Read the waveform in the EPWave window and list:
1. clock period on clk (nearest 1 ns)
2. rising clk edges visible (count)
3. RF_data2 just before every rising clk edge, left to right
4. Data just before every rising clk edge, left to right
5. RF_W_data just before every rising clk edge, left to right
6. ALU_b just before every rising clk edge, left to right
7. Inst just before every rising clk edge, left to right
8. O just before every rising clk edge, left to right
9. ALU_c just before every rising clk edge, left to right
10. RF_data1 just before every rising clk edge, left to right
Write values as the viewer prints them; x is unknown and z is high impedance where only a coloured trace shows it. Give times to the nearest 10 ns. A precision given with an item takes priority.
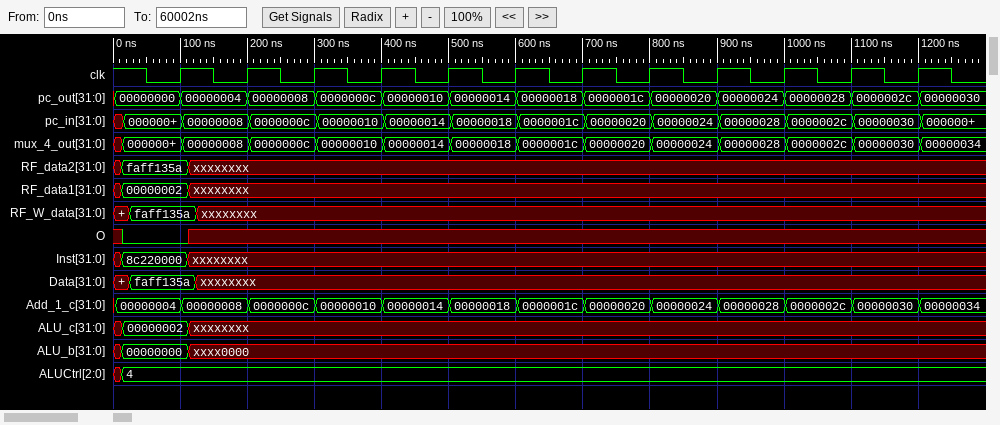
100 ns
12
faff135a, xxxxxxxx, xxxxxxxx, xxxxxxxx, xxxxxxxx, xxxxxxxx, xxxxxxxx, xxxxxxxx, xxxxxxxx, xxxxxxxx, xxxxxxxx, xxxxxxxx
faff135a, xxxxxxxx, xxxxxxxx, xxxxxxxx, xxxxxxxx, xxxxxxxx, xxxxxxxx, xxxxxxxx, xxxxxxxx, xxxxxxxx, xxxxxxxx, xxxxxxxx
faff135a, xxxxxxxx, xxxxxxxx, xxxxxxxx, xxxxxxxx, xxxxxxxx, xxxxxxxx, xxxxxxxx, xxxxxxxx, xxxxxxxx, xxxxxxxx, xxxxxxxx
00000000, xxxx0000, xxxx0000, xxxx0000, xxxx0000, xxxx0000, xxxx0000, xxxx0000, xxxx0000, xxxx0000, xxxx0000, xxxx0000
8c220000, xxxxxxxx, xxxxxxxx, xxxxxxxx, xxxxxxxx, xxxxxxxx, xxxxxxxx, xxxxxxxx, xxxxxxxx, xxxxxxxx, xxxxxxxx, xxxxxxxx
0 x x x x x x x x x x x
00000002, xxxxxxxx, xxxxxxxx, xxxxxxxx, xxxxxxxx, xxxxxxxx, xxxxxxxx, xxxxxxxx, xxxxxxxx, xxxxxxxx, xxxxxxxx, xxxxxxxx
00000002, xxxxxxxx, xxxxxxxx, xxxxxxxx, xxxxxxxx, xxxxxxxx, xxxxxxxx, xxxxxxxx, xxxxxxxx, xxxxxxxx, xxxxxxxx, xxxxxxxx
